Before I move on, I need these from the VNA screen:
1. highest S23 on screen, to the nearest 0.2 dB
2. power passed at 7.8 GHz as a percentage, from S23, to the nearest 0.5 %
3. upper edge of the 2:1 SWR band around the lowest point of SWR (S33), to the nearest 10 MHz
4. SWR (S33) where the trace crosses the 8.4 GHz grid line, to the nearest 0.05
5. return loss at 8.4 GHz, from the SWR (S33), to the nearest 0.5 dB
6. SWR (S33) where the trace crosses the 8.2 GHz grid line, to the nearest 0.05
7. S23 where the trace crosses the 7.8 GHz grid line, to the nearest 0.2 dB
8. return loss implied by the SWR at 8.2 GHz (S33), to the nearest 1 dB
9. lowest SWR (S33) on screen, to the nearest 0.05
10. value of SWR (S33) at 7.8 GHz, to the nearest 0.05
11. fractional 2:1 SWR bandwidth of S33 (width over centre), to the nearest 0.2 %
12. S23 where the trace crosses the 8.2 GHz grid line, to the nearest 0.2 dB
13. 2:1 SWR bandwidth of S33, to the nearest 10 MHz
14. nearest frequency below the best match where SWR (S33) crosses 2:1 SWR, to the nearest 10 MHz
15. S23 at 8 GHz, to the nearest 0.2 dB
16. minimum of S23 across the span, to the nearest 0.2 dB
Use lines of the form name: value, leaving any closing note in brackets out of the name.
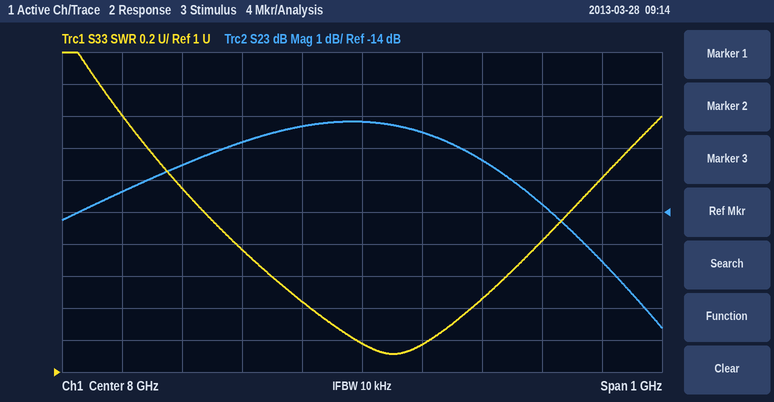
highest S23 on screen, to the nearest 0.2 dB: -11.2 dB
power passed at 7.8 GHz as a percentage, from S23, to the nearest 0.5 %: 6.5 %
upper edge of the 2:1 SWR band around the lowest point of SWR (S33), to the nearest 10 MHz: 8.35 GHz
SWR (S33) where the trace crosses the 8.4 GHz grid line, to the nearest 0.05: 2.20
return loss at 8.4 GHz, from the SWR (S33), to the nearest 0.5 dB: 8.5 dB
SWR (S33) where the trace crosses the 8.2 GHz grid line, to the nearest 0.05: 1.45
S23 where the trace crosses the 7.8 GHz grid line, to the nearest 0.2 dB: -11.8 dB
return loss implied by the SWR at 8.2 GHz (S33), to the nearest 1 dB: 15 dB
lowest SWR (S33) on screen, to the nearest 0.05: 1.10
value of SWR (S33) at 7.8 GHz, to the nearest 0.05: 1.75
fractional 2:1 SWR bandwidth of S33 (width over centre), to the nearest 0.2 %: 7.6 %
S23 where the trace crosses the 8.2 GHz grid line, to the nearest 0.2 dB: -12.4 dB
2:1 SWR bandwidth of S33, to the nearest 10 MHz: 610 MHz
nearest frequency below the best match where SWR (S33) crosses 2:1 SWR, to the nearest 10 MHz: 7.74 GHz
S23 at 8 GHz, to the nearest 0.2 dB: -11.2 dB
minimum of S23 across the span, to the nearest 0.2 dB: -17.6 dB
